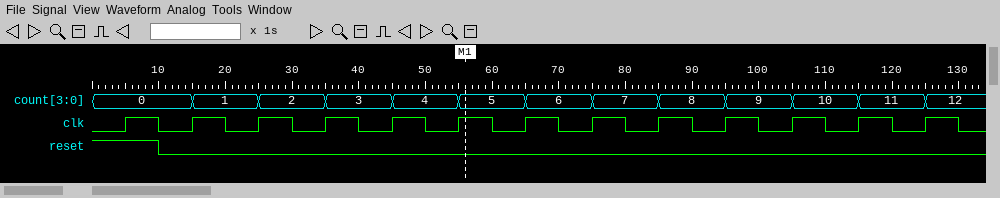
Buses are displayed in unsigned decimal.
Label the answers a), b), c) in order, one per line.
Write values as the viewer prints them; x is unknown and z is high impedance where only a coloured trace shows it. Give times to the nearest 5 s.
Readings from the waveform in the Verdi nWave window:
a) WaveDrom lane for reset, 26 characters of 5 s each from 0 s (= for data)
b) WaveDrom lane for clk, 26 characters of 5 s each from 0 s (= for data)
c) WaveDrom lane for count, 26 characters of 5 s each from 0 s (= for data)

a) {name: 'reset', wave: '1.0.......................'}
b) {name: 'clk', wave: '01010101010101010101010101'}
c) {name: 'count', wave: '=..=.=.=.=.=.=.=.=.=.=.=.=', data: '0 1 2 3 4 5 6 7 8 9 10 11 12'}
